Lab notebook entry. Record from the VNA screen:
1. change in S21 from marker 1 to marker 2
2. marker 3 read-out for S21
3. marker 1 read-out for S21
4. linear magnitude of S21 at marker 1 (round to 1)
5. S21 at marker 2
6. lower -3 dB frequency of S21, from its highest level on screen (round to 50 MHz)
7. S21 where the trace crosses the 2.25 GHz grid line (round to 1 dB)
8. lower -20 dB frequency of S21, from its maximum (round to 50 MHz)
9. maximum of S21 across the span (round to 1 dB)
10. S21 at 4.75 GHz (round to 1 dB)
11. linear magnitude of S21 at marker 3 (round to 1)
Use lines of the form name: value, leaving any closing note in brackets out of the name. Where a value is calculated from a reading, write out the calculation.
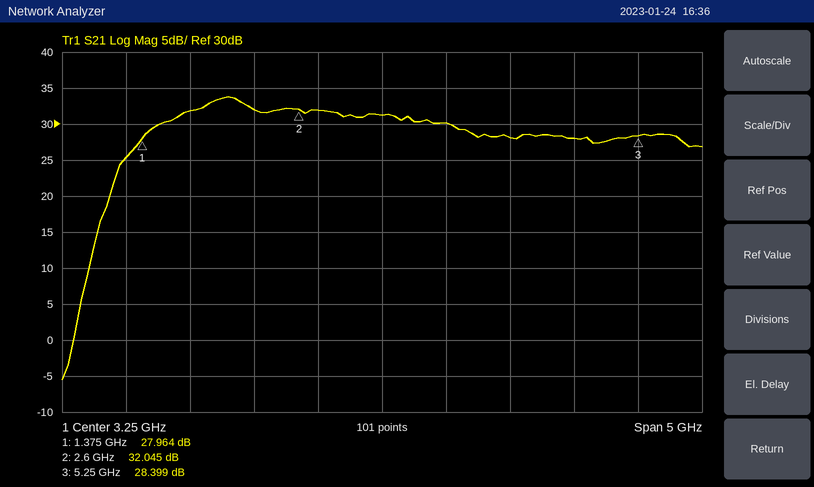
change in S21 from marker 1 to marker 2: 32.045 − (27.964) = 4.081 dB
marker 3 read-out for S21: 28.399 dB
marker 1 read-out for S21: 27.964 dB
linear magnitude of S21 at marker 1: 10^(27.964/20) ≈ 25
S21 at marker 2: 32.045 dB
lower -3 dB frequency of S21, from its highest level on screen: 1.65 GHz
S21 where the trace crosses the 2.25 GHz grid line: 32 dB
lower -20 dB frequency of S21, from its maximum: 1.00 GHz
maximum of S21 across the span: 34 dB
S21 at 4.75 GHz: 28 dB
linear magnitude of S21 at marker 3: 10^(28.399/20) ≈ 26
